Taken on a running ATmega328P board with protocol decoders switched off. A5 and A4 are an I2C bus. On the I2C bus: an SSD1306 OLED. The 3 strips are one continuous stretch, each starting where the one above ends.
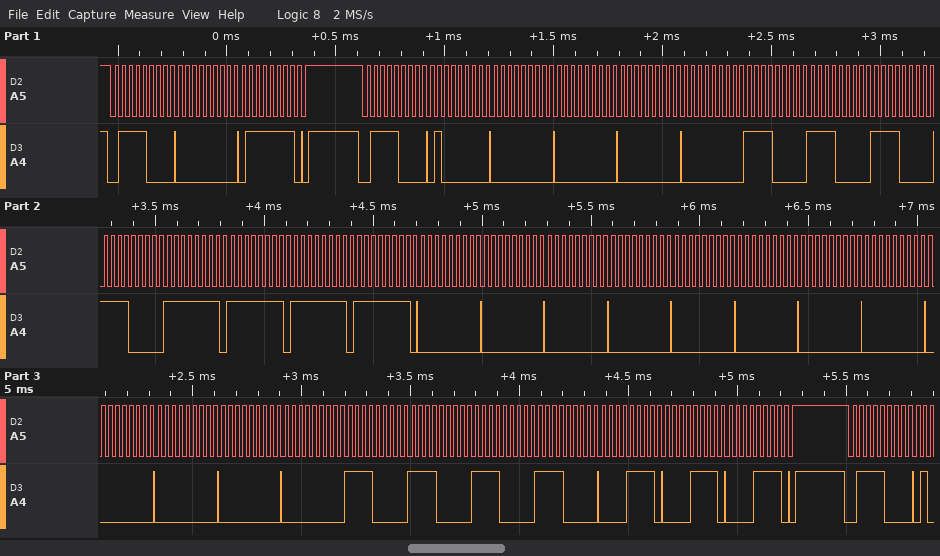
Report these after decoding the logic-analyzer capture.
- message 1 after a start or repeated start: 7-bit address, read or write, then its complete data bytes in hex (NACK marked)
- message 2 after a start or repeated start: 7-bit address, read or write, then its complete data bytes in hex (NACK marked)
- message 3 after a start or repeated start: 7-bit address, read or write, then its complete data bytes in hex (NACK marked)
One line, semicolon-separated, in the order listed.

0x3C write: 00 7F; 0x3C write: 40 00 00 00 00 F0 F0 F0 F0 FF FF FF FF 00 00 00 00 00 00 00 00 00 00 00 00 F0 F0 F0 F0 0F 0F 0F; 0x3C write
